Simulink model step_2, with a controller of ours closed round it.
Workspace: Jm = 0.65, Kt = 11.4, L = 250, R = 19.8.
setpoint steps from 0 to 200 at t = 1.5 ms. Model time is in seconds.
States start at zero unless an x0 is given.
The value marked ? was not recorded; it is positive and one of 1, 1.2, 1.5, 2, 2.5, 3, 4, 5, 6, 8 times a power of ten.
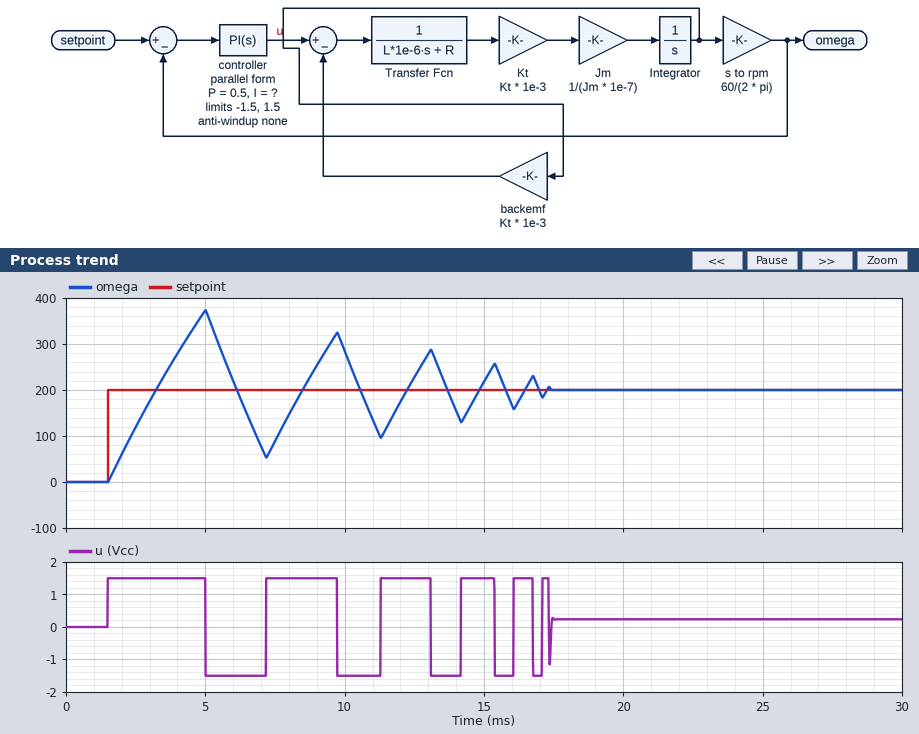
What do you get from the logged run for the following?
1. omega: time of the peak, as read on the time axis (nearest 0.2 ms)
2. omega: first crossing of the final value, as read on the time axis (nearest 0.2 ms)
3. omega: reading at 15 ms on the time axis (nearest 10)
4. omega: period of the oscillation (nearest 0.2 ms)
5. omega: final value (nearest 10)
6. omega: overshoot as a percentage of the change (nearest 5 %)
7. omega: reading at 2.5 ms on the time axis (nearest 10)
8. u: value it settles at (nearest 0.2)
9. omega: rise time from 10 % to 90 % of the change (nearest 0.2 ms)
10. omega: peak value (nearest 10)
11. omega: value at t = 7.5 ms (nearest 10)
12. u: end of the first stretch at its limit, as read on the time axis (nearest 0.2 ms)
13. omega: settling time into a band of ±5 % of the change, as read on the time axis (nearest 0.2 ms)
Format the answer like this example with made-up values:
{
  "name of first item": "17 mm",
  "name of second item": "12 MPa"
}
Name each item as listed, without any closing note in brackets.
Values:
{
  "omega: time of the peak, as read on the time axis": "5.0 ms",
  "omega: first crossing of the final value, as read on the time axis": "3.2 ms",
  "omega: reading at 15 ms on the time axis": "220",
  "omega: period of the oscillation": "4.8 ms",
  "omega: final value": "200",
  "omega: overshoot as a percentage of the change": "85 %",
  "omega: reading at 2.5 ms on the time axis": "120",
  "u: value it settles at": "0.2",
  "omega: rise time from 10 % to 90 % of the change": "1.4 ms",
  "omega: peak value": "370",
  "omega: value at t = 7.5 ms": "90",
  "u: end of the first stretch at its limit, as read on the time axis": "5.0 ms",
  "omega: settling time into a band of ±5 % of the change, as read on the time axis": "17.2 ms"
}
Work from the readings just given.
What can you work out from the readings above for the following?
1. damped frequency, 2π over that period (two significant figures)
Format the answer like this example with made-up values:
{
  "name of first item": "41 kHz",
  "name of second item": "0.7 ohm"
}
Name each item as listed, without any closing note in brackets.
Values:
{
  "damped frequency, 2π over that period": "1.3 rad/ms"
}
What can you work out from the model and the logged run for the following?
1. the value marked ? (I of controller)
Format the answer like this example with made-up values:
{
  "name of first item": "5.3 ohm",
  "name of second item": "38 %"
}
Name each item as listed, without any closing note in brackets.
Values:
{
  "the value marked ?": "8000"
}
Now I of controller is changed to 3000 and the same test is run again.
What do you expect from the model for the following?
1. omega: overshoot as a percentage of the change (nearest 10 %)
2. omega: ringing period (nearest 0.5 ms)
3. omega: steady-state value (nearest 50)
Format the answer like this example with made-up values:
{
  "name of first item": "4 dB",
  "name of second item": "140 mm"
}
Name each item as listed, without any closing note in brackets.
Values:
{
  "omega: overshoot as a percentage of the change": "80 %",
  "omega: ringing period": "3.5 ms",
  "omega: steady-state value": "200"
}
